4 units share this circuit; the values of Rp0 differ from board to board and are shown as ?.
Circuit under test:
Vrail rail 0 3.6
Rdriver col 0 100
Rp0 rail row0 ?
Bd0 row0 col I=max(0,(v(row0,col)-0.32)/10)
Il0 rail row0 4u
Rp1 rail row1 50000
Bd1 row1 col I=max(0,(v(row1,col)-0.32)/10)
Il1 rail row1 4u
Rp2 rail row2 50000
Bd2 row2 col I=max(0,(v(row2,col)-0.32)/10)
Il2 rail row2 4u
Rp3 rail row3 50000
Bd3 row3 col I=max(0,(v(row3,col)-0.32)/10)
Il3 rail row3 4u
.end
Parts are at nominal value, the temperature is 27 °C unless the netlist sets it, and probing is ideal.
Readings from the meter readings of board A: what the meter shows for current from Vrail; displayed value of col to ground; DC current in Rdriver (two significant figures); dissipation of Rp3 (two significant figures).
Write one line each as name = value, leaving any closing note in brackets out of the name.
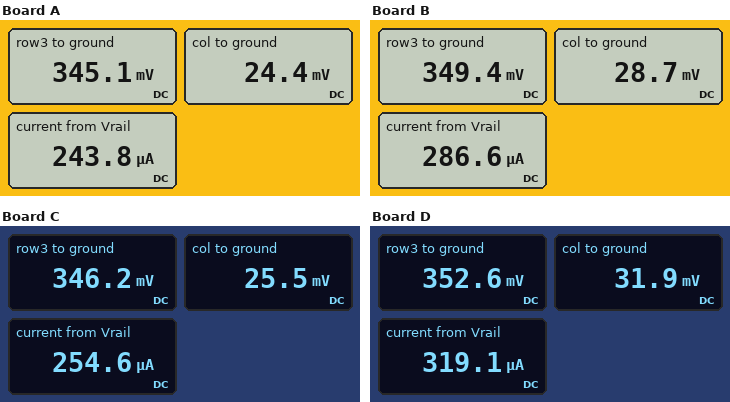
what the meter shows for current from Vrail = 243.8 µA
displayed value of col to ground = 24.4 mV
DC current in Rdriver = 240 µA
dissipation of Rp3 = 210 µW
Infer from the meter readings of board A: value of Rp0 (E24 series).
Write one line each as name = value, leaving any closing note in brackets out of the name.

value of Rp0 = 100 kΩ
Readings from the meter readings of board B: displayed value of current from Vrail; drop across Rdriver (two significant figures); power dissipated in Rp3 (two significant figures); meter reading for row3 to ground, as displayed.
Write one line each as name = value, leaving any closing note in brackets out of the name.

displayed value of current from Vrail = 286.6 µA
drop across Rdriver = 29 mV
power dissipated in Rp3 = 210 µW
meter reading for row3 to ground, as displayed = 349.4 mV
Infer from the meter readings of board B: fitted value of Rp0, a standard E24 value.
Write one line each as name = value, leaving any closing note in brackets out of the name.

fitted value of Rp0, a standard E24 value = 43 kΩ
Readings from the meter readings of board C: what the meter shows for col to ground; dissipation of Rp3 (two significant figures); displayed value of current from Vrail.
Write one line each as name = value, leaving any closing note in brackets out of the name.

what the meter shows for col to ground = 25.5 mV
dissipation of Rp3 = 210 µW
displayed value of current from Vrail = 254.6 µA
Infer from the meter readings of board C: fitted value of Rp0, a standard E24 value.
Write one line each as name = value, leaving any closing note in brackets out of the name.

fitted value of Rp0, a standard E24 value = 75 kΩ
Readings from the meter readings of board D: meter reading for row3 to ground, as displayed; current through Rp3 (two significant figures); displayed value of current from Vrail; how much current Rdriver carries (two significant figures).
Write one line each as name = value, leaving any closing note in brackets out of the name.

meter reading for row3 to ground, as displayed = 352.6 mV
current through Rp3 = 65 µA
displayed value of current from Vrail = 319.1 µA
how much current Rdriver carries = 320 µA
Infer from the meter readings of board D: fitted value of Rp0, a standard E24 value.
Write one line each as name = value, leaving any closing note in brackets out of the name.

fitted value of Rp0, a standard E24 value = 30 kΩ
